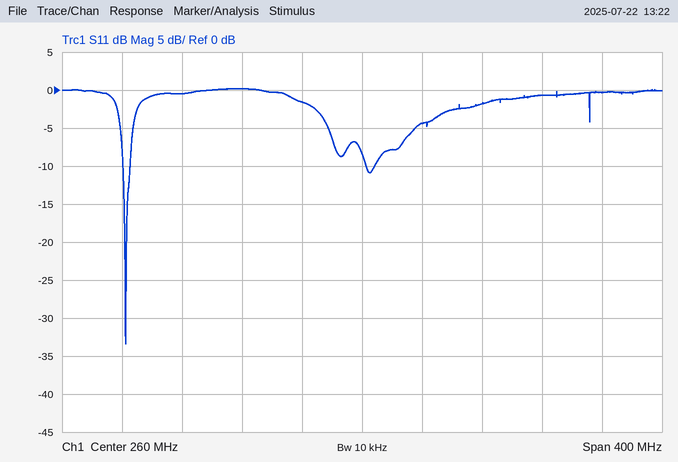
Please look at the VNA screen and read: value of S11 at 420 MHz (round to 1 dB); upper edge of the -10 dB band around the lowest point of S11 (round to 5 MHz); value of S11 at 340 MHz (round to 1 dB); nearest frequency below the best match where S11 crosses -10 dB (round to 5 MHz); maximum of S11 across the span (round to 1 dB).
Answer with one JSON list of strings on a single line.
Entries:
["0 dB", "105 MHz", "-2 dB", "100 MHz", "0 dB"]
